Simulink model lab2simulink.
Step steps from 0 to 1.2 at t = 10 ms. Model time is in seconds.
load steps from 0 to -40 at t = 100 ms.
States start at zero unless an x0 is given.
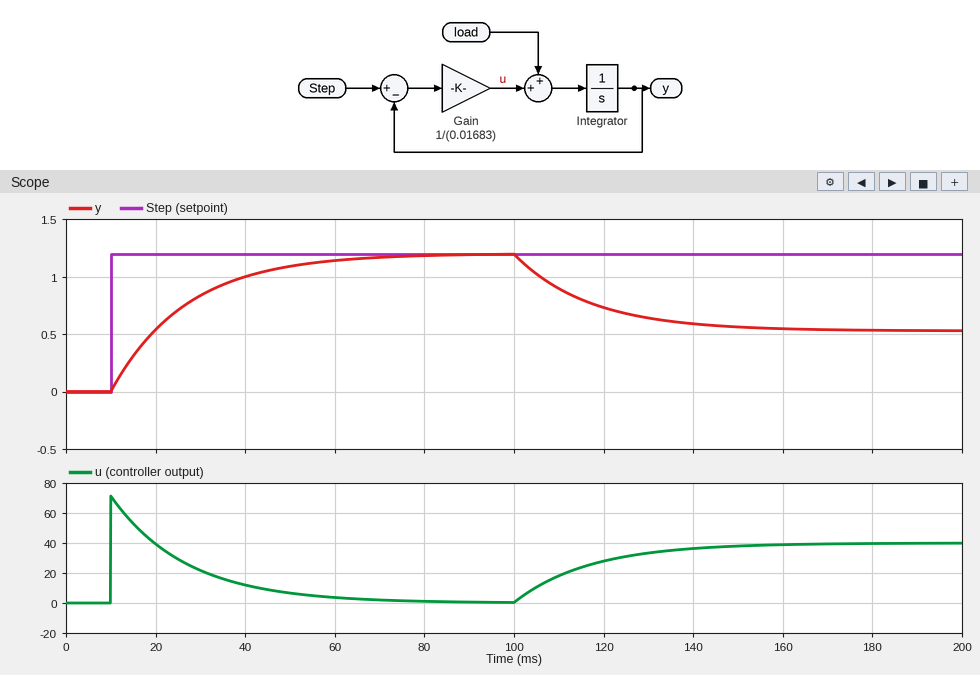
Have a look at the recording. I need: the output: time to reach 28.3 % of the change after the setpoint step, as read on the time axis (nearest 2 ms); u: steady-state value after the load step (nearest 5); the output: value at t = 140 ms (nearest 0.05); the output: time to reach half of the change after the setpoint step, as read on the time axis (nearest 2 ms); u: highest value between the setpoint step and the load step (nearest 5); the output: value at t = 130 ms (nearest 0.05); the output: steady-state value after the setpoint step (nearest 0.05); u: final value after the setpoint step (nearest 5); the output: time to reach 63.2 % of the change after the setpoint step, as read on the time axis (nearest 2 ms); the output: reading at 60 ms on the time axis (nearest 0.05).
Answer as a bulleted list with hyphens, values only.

- 16 ms
- 40
- 0.60
- 22 ms
- 70
- 0.65
- 1.20
- 0
- 26 ms
- 1.15
